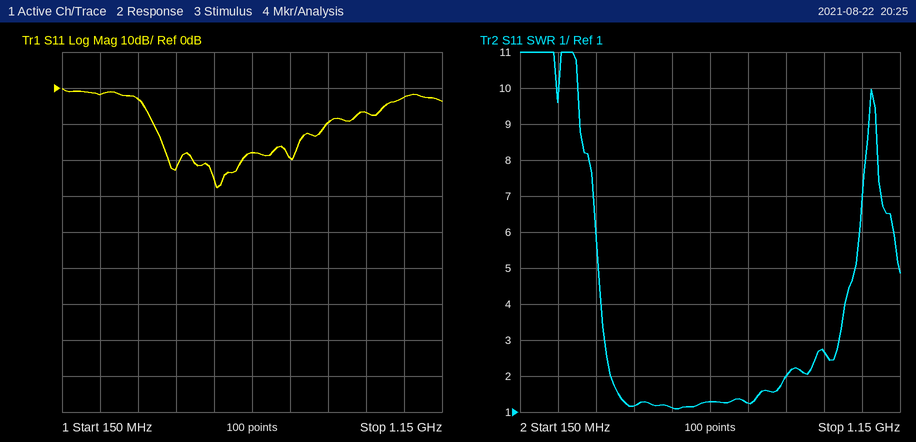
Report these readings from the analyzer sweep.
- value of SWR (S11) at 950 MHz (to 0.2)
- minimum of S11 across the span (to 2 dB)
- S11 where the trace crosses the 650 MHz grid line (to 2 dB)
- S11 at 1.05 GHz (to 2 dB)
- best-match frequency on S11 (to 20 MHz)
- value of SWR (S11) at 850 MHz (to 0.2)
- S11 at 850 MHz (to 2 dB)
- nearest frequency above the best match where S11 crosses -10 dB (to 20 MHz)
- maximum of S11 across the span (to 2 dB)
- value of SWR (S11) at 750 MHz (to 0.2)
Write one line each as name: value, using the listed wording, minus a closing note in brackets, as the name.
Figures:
value of SWR (S11) at 950 MHz: 2.6
minimum of S11 across the span: -28 dB
S11 where the trace crosses the 650 MHz grid line: -18 dB
S11 at 1.05 GHz: -2 dB
best-match frequency on S11: 560 MHz
value of SWR (S11) at 850 MHz: 2.0
S11 at 850 MHz: -10 dB
nearest frequency above the best match where S11 crosses -10 dB: 840 MHz
maximum of S11 across the span: 0 dB
value of SWR (S11) at 750 MHz: 1.2
